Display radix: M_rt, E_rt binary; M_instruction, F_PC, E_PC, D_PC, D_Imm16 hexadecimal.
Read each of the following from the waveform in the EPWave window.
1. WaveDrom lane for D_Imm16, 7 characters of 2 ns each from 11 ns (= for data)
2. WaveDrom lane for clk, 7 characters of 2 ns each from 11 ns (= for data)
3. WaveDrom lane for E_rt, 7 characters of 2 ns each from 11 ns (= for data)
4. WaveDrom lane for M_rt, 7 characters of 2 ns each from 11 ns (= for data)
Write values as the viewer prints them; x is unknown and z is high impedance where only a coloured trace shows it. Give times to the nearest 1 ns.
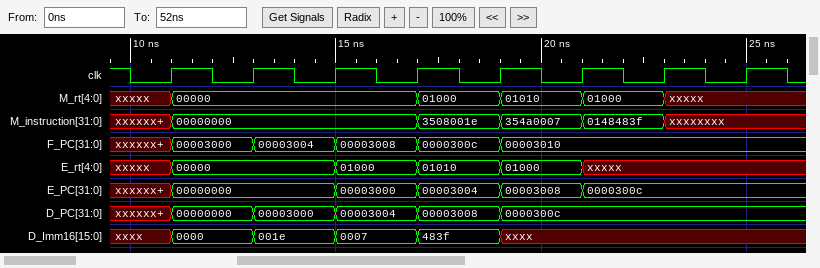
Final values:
{name: 'D_Imm16', wave: '====x..', data: '0000 001e 0007 483f'}
{name: 'clk', wave: 'p......'}
{name: 'E_rt', wave: '=.===x.', data: '00000 01000 01010 01000'}
{name: 'M_rt', wave: '=..===x', data: '00000 01000 01010 01000'}
